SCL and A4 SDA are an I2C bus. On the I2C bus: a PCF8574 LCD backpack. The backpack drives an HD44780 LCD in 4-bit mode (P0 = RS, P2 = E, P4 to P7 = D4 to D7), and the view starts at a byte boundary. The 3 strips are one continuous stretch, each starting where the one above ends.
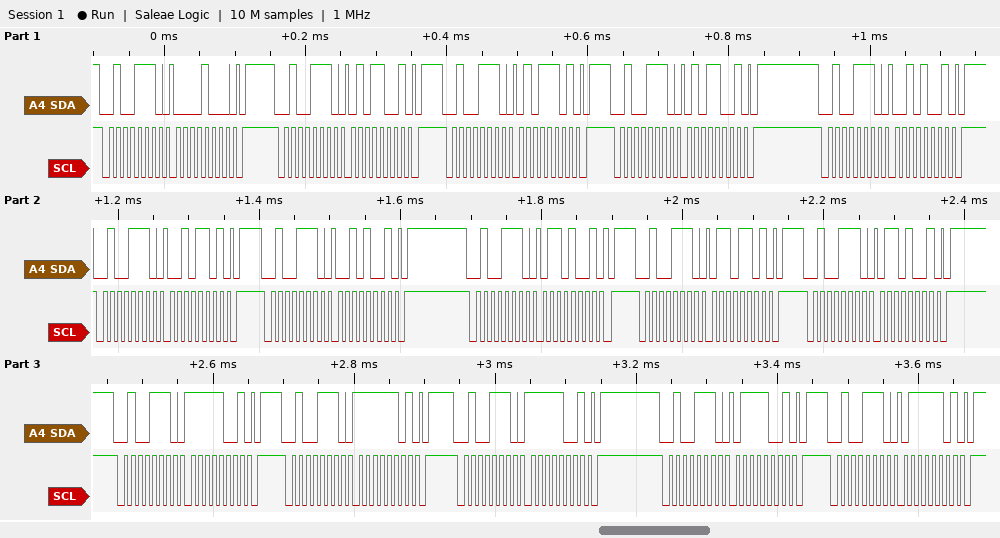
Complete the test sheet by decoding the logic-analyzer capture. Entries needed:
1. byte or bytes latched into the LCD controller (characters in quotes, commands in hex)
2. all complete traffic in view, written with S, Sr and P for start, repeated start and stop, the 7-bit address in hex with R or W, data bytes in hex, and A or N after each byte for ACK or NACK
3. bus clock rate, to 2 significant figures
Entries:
'R' 'o'
S 27W A 08 A P S 27W A 59 A P S 27W A 5D A P S 27W A 59 A P S 27W A 29 A P S 27W A 2D A P S 27W A 29 A P S 27W A 69 A P S 27W A 6D A P S 27W A 69 A P S 27W A F9 A P S 27W A FD A P S 27W A F9 A P S 27W A 79 A P S 27W A 7D A P
100 kHz
